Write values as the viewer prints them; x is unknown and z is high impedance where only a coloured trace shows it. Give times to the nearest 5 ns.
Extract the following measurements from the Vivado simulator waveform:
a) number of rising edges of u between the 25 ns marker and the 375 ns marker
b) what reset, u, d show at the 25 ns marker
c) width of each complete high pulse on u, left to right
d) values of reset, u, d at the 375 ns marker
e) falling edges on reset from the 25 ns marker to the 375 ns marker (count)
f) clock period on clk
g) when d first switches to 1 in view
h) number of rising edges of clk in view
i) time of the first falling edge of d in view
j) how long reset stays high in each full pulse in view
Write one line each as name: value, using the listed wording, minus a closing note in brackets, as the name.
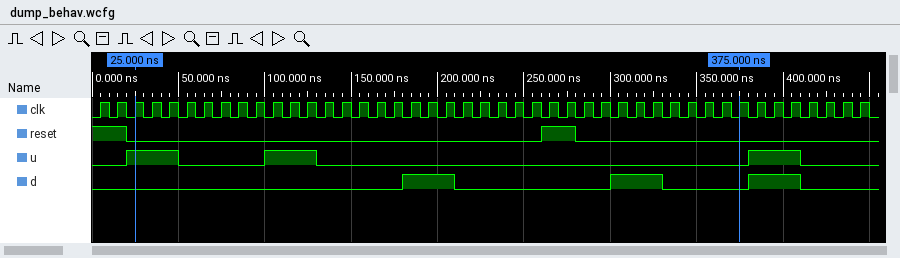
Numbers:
number of rising edges of u between the 25 ns marker and the 375 ns marker: 1
what reset, u, d show at the 25 ns marker: reset=0, u=1, d=0
width of each complete high pulse on u, left to right: 30 ns, 30 ns, 30 ns
values of reset, u, d at the 375 ns marker: reset=0, u=0, d=0
falling edges on reset from the 25 ns marker to the 375 ns marker: 1
clock period on clk: 10 ns
when d first switches to 1 in view: 180 ns
number of rising edges of clk in view: 45
time of the first falling edge of d in view: 210 ns
how long reset stays high in each full pulse in view: 20 ns
